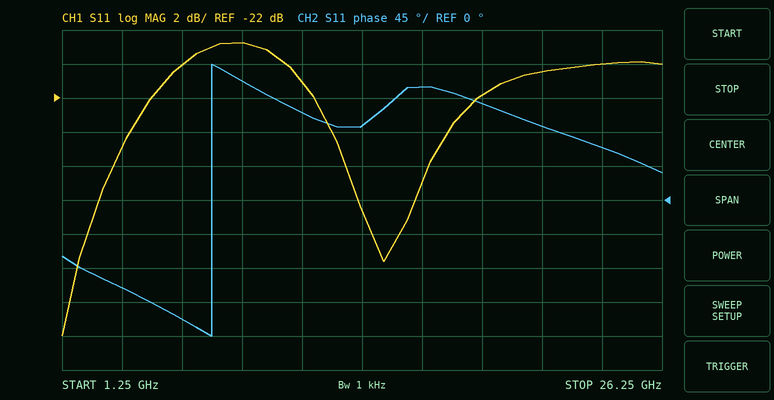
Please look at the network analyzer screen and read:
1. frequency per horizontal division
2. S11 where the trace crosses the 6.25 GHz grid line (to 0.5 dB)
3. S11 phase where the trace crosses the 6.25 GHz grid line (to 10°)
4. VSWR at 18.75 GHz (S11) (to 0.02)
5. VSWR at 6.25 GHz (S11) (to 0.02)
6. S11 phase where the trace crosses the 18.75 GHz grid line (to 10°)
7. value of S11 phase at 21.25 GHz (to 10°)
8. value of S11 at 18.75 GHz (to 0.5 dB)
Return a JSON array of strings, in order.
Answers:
["2.5 GHz", "-20.0 dB", "-160°", "1.18", "1.22", "130°", "100°", "-22.0 dB"]
